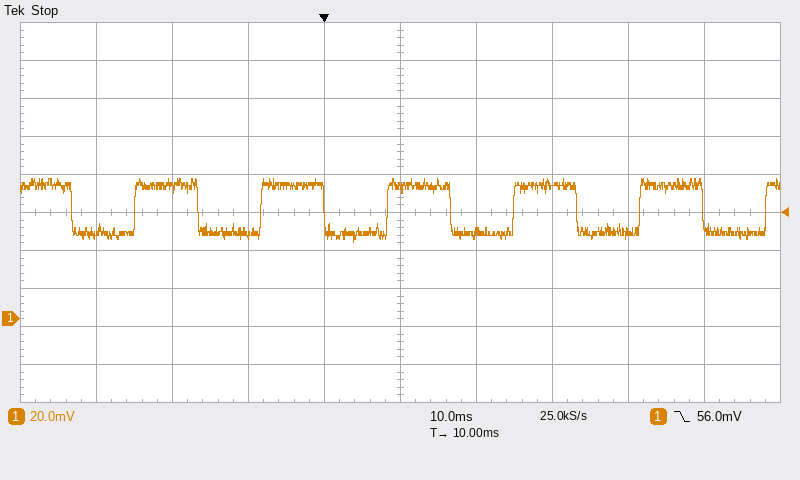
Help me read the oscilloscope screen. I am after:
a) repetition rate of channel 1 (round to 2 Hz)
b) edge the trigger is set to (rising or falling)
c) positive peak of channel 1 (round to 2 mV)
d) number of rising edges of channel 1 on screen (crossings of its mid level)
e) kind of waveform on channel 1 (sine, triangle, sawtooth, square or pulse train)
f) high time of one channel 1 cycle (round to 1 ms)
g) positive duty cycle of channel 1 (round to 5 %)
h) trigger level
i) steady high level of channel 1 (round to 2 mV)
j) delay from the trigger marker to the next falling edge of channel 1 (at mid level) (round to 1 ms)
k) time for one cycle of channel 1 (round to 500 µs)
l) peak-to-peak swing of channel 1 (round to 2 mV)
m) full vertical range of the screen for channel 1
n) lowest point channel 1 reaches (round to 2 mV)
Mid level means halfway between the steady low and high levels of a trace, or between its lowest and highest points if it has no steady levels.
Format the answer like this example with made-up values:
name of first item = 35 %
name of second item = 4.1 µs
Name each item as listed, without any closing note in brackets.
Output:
repetition rate of channel 1 = 60 Hz
edge the trigger is set to = falling
positive peak of channel 1 = 74 mV
number of rising edges of channel 1 on screen = 6
kind of waveform on channel 1 = square
high time of one channel 1 cycle = 8 ms
positive duty cycle of channel 1 = 50 %
trigger level = 56.0 mV
steady high level of channel 1 = 70 mV
delay from the trigger marker to the next falling edge of channel 1 (at mid level) = 17 ms
time for one cycle of channel 1 = 16.5 ms
peak-to-peak swing of channel 1 = 34 mV
full vertical range of the screen for channel 1 = 200 mV
lowest point channel 1 reaches = 40 mV
